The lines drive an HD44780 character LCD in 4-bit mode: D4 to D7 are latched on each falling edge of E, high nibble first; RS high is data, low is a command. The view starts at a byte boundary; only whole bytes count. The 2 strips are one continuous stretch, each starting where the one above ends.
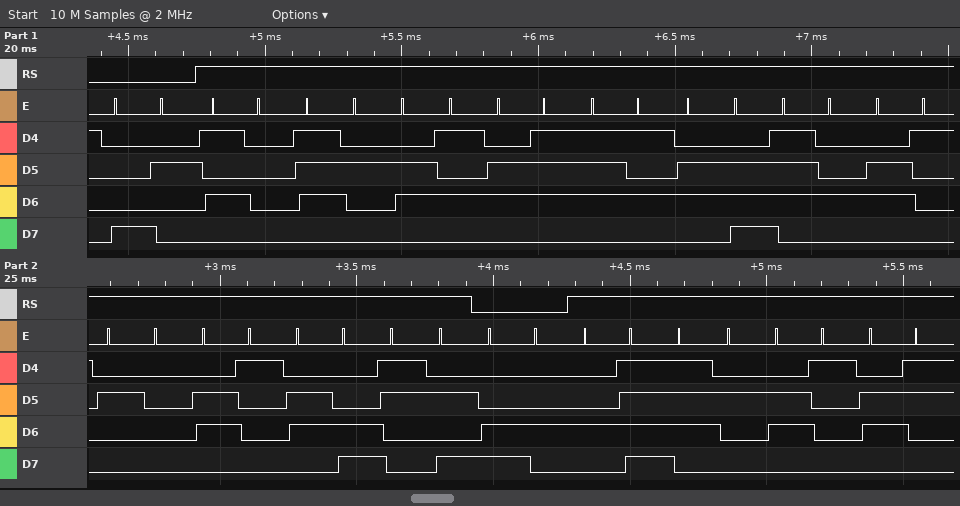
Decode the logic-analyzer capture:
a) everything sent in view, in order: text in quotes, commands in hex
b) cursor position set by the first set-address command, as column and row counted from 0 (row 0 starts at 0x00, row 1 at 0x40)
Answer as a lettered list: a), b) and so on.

a) 0x82 "Pregunta al:" 0xC4 "Orac"
b) column 2, row 0
